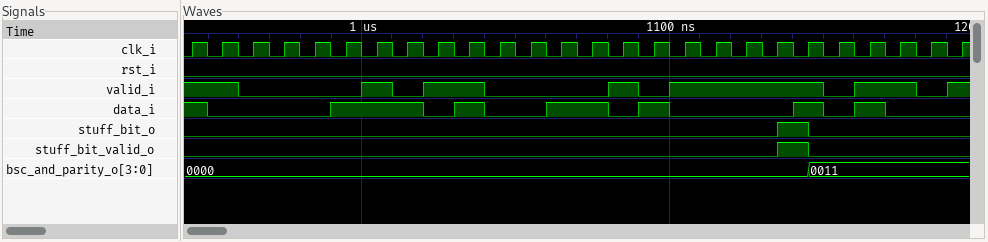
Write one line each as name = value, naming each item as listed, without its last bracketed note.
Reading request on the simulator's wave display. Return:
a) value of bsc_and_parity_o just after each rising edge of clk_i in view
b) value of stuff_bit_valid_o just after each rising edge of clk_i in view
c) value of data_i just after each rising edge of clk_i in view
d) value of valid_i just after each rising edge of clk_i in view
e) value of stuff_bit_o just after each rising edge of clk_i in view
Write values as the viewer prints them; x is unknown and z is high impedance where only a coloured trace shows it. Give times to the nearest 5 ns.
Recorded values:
value of bsc_and_parity_o just after each rising edge of clk_i in view = 0000, 0000, 0000, 0000, 0000, 0000, 0000, 0000, 0000, 0000, 0000, 0000, 0000, 0000, 0000, 0000, 0000, 0000, 0000, 0000, 0011, 0011, 0011, 0011, 0011, 0011
value of stuff_bit_valid_o just after each rising edge of clk_i in view = 0 0 0 0 0 0 0 0 0 0 0 0 0 0 0 0 0 0 0 1 0 0 0 0 0 0
value of data_i just after each rising edge of clk_i in view = 1 0 0 0 0 1 1 1 0 1 0 0 1 1 0 1 0 0 0 0 1 0 1 0 0 0
value of valid_i just after each rising edge of clk_i in view = 1 1 0 0 0 0 1 0 1 1 0 0 0 0 1 0 1 1 1 1 1 0 1 1 0 1
value of stuff_bit_o just after each rising edge of clk_i in view = 0 0 0 0 0 0 0 0 0 0 0 0 0 0 0 0 0 0 0 1 0 0 0 0 0 0
